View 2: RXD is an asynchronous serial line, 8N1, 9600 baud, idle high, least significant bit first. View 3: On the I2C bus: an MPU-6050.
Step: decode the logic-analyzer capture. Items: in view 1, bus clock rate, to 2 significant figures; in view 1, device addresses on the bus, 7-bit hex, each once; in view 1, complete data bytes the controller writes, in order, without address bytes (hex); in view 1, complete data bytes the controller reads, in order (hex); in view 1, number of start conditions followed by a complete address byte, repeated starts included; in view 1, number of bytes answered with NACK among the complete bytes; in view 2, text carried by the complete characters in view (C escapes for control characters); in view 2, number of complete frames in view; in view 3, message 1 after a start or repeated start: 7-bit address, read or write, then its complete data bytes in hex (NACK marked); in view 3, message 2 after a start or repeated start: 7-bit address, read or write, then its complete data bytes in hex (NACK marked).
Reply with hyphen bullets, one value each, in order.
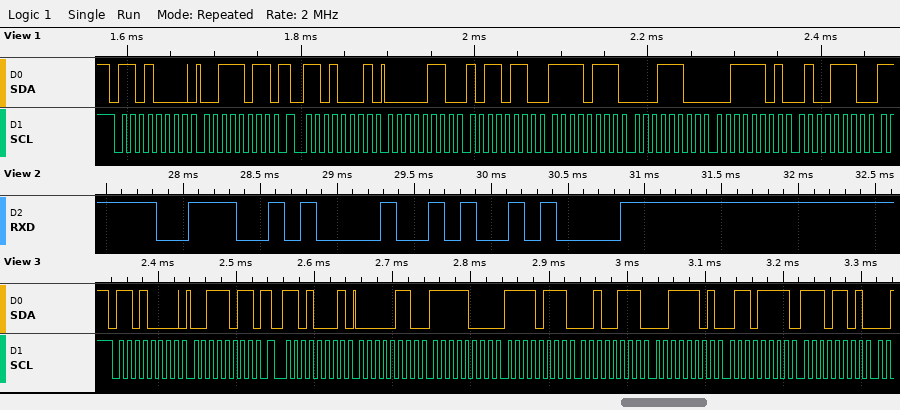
- 100 kHz
- 0x68
- 3B
- 06 B6 F7 1C 3D 4E
- 2
- 0
- "NH\n"
- 3
- 0x68 write: 3B
- 0x68 read: 06 F8 F7 27 3D 6F ED
